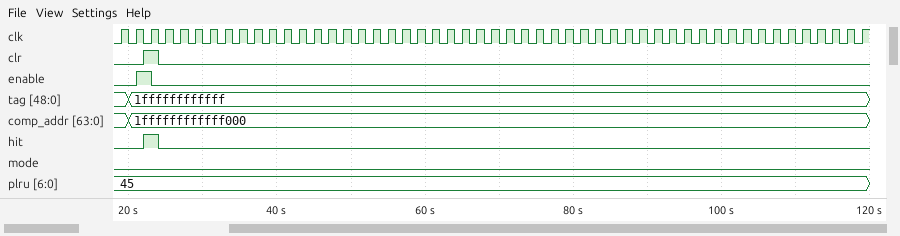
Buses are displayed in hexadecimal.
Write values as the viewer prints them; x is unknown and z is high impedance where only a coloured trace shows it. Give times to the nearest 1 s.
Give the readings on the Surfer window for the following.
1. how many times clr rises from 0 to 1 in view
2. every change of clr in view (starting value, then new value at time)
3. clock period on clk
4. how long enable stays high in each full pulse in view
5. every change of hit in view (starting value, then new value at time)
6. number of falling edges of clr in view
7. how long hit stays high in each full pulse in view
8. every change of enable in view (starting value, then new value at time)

1
0, 1 at 22 s, 0 at 24 s
2 s
2 s
0, 1 at 22 s, 0 at 24 s
1
2 s
0, 1 at 21 s, 0 at 23 s
